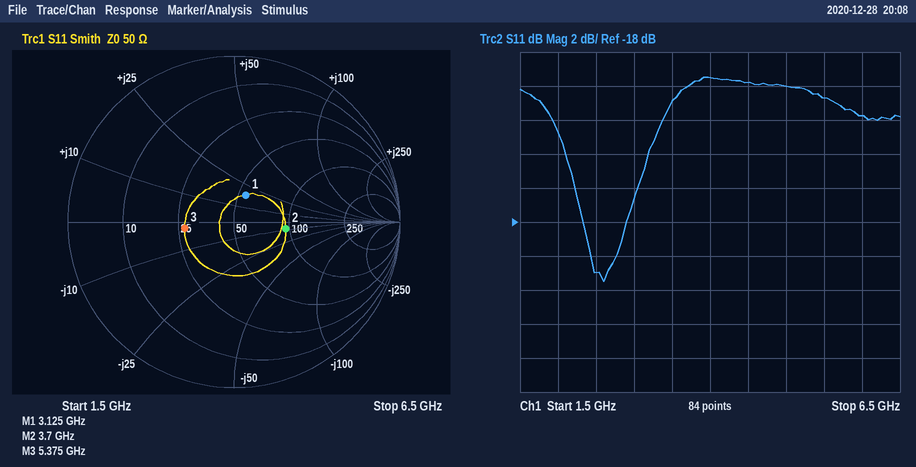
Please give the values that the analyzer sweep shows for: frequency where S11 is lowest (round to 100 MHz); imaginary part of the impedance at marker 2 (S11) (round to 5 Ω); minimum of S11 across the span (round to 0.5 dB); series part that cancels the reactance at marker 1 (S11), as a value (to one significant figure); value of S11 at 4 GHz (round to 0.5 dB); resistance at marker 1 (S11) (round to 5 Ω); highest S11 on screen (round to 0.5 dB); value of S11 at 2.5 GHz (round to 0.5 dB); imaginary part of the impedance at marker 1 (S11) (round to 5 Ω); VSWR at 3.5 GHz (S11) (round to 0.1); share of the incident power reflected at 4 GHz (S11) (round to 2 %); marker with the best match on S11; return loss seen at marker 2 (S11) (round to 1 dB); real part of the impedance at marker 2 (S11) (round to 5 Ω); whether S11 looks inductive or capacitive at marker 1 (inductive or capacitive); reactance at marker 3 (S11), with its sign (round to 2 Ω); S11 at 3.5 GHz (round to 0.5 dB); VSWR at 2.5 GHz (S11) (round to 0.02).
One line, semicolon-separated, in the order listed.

2.6 GHz; -10 Ω; -21.5 dB; 3 pF; -9.5 dB; 55 Ω; -9.5 dB; -21.0 dB; +20 Ω; 1.8; 12 %; marker 1; 10 dB; 95 Ω; inductive; -2 Ω; -11.0 dB; 1.20
